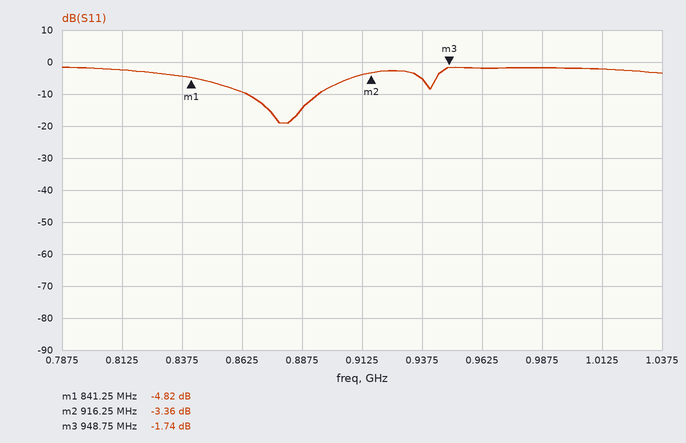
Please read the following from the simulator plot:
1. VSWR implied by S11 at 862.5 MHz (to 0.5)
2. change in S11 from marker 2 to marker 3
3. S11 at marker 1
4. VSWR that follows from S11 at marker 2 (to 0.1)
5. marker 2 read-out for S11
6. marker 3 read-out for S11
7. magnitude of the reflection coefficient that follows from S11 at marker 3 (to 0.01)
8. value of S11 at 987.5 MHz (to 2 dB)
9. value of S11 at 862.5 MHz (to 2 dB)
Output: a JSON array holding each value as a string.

["2.0", "1.62 dB", "-4.82 dB", "5.2", "-3.36 dB", "-1.74 dB", "0.82", "-2 dB", "-10 dB"]
